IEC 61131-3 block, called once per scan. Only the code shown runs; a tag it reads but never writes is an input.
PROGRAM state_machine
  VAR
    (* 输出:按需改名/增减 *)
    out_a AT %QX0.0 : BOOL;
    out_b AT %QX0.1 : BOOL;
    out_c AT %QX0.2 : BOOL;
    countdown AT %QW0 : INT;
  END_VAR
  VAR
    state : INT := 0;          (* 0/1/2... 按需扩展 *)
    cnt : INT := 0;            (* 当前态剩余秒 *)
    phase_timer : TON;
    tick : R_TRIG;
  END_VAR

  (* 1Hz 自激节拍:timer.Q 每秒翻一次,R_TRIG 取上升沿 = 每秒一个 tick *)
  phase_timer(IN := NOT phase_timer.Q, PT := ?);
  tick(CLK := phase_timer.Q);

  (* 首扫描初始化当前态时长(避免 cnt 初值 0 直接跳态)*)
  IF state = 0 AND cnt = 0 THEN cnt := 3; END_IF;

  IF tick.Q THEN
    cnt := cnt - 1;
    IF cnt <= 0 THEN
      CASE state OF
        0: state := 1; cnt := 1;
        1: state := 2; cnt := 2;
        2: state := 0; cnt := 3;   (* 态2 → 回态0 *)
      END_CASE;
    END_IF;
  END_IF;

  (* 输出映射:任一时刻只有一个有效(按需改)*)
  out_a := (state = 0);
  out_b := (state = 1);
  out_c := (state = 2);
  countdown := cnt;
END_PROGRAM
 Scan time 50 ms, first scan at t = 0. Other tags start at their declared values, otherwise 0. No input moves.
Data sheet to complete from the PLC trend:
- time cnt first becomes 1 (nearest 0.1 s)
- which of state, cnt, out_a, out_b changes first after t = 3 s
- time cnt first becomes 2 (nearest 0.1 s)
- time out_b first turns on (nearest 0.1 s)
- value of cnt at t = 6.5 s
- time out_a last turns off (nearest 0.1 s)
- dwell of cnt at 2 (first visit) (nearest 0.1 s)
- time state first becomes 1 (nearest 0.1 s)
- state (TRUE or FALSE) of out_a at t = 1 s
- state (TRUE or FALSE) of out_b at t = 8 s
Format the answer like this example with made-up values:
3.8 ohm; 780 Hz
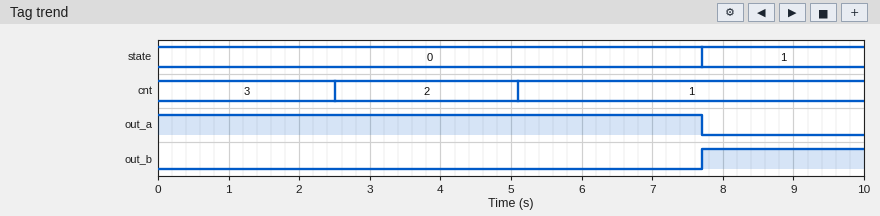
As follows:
5.1 s; cnt; 2.5 s; 7.7 s; 1; 7.7 s; 2.6 s; 7.7 s; TRUE; TRUE
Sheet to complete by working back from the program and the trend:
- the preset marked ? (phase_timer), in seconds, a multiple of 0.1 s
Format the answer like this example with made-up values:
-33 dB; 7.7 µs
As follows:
2.5 s
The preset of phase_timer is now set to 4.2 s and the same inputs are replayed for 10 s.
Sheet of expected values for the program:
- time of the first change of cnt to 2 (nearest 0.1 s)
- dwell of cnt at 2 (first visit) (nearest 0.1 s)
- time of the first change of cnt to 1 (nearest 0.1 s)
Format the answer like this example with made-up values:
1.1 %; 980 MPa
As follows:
4.2 s; 4.3 s; 8.5 s
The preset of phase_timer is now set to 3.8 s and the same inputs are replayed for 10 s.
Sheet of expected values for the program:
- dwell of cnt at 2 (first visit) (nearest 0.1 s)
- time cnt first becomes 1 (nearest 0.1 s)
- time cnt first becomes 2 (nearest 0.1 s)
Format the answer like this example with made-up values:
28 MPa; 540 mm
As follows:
3.9 s; 7.7 s; 3.8 s
